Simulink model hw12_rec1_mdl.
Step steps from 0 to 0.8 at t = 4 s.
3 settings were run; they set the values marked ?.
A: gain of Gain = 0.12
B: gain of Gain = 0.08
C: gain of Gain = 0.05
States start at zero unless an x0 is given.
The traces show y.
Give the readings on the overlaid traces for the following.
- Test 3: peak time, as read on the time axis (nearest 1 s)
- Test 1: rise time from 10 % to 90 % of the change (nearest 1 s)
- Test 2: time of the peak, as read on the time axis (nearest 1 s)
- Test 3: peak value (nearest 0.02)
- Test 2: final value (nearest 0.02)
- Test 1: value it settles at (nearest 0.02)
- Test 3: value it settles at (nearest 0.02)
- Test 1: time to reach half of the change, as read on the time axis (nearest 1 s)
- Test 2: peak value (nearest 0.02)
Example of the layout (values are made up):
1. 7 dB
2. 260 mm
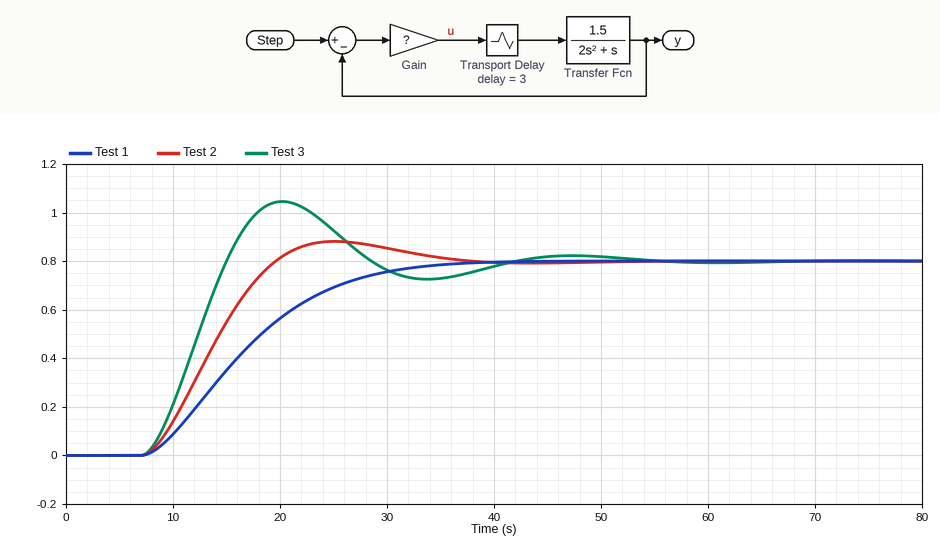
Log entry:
1. 20 s
2. 17 s
3. 25 s
4. 1.04
5. 0.80
6. 0.80
7. 0.80
8. 16 s
9. 0.88
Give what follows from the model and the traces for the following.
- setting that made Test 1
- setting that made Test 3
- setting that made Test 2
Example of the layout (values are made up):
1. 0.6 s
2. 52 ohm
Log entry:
1. C
2. A
3. B
